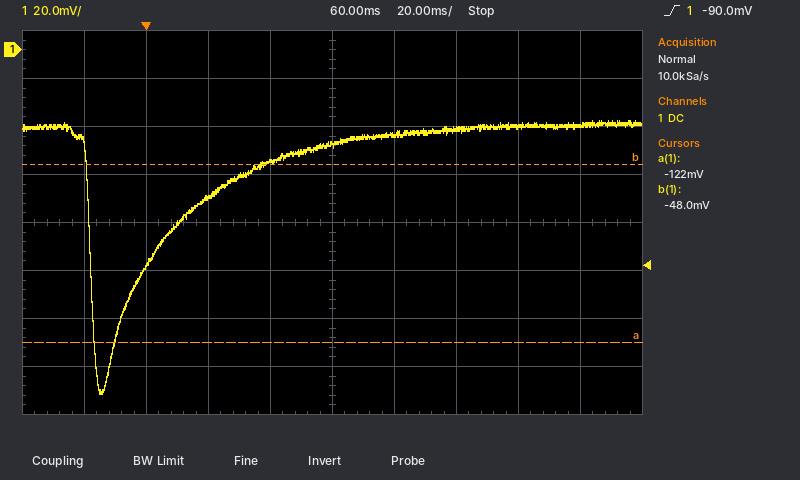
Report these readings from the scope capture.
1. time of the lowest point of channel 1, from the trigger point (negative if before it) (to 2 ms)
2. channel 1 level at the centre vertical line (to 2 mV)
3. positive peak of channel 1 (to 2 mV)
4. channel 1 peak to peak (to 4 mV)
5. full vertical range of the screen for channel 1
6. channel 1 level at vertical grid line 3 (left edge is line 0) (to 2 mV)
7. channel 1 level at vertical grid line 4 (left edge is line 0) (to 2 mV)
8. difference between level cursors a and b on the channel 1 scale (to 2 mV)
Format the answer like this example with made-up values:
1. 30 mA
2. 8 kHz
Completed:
1. -14 ms
2. -40 mV
3. -30 mV
4. 112 mV
5. 160 mV
6. -62 mV
7. -46 mV
8. 74 mV
